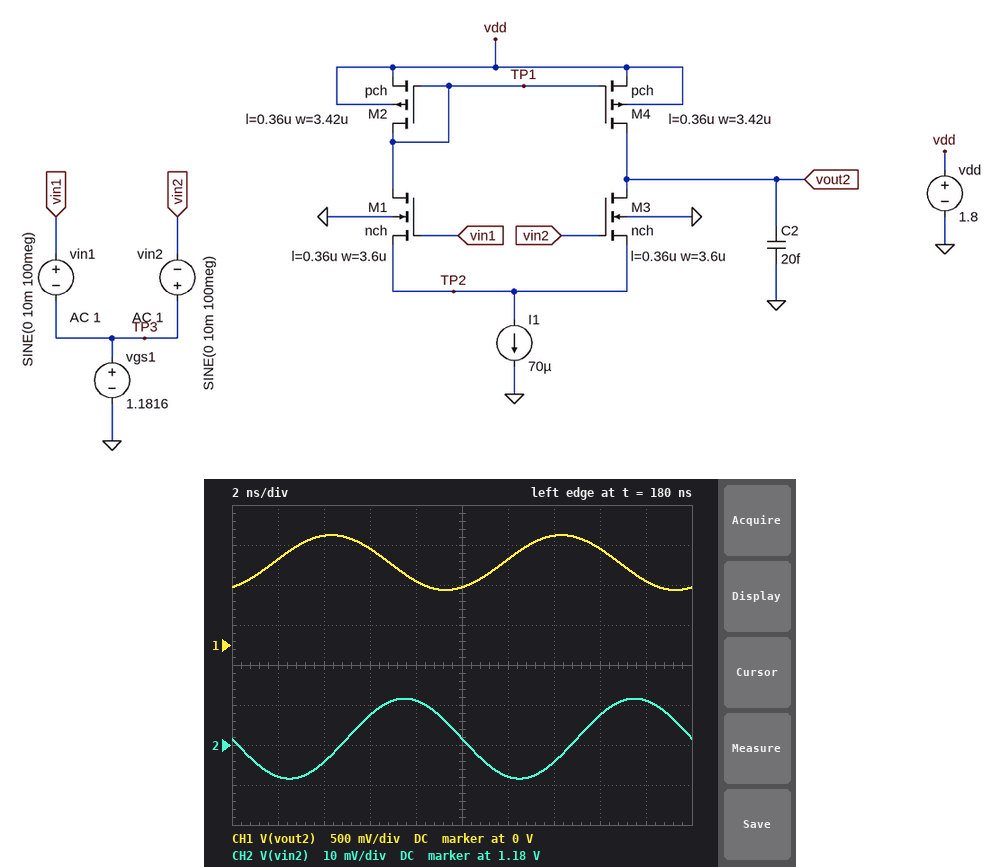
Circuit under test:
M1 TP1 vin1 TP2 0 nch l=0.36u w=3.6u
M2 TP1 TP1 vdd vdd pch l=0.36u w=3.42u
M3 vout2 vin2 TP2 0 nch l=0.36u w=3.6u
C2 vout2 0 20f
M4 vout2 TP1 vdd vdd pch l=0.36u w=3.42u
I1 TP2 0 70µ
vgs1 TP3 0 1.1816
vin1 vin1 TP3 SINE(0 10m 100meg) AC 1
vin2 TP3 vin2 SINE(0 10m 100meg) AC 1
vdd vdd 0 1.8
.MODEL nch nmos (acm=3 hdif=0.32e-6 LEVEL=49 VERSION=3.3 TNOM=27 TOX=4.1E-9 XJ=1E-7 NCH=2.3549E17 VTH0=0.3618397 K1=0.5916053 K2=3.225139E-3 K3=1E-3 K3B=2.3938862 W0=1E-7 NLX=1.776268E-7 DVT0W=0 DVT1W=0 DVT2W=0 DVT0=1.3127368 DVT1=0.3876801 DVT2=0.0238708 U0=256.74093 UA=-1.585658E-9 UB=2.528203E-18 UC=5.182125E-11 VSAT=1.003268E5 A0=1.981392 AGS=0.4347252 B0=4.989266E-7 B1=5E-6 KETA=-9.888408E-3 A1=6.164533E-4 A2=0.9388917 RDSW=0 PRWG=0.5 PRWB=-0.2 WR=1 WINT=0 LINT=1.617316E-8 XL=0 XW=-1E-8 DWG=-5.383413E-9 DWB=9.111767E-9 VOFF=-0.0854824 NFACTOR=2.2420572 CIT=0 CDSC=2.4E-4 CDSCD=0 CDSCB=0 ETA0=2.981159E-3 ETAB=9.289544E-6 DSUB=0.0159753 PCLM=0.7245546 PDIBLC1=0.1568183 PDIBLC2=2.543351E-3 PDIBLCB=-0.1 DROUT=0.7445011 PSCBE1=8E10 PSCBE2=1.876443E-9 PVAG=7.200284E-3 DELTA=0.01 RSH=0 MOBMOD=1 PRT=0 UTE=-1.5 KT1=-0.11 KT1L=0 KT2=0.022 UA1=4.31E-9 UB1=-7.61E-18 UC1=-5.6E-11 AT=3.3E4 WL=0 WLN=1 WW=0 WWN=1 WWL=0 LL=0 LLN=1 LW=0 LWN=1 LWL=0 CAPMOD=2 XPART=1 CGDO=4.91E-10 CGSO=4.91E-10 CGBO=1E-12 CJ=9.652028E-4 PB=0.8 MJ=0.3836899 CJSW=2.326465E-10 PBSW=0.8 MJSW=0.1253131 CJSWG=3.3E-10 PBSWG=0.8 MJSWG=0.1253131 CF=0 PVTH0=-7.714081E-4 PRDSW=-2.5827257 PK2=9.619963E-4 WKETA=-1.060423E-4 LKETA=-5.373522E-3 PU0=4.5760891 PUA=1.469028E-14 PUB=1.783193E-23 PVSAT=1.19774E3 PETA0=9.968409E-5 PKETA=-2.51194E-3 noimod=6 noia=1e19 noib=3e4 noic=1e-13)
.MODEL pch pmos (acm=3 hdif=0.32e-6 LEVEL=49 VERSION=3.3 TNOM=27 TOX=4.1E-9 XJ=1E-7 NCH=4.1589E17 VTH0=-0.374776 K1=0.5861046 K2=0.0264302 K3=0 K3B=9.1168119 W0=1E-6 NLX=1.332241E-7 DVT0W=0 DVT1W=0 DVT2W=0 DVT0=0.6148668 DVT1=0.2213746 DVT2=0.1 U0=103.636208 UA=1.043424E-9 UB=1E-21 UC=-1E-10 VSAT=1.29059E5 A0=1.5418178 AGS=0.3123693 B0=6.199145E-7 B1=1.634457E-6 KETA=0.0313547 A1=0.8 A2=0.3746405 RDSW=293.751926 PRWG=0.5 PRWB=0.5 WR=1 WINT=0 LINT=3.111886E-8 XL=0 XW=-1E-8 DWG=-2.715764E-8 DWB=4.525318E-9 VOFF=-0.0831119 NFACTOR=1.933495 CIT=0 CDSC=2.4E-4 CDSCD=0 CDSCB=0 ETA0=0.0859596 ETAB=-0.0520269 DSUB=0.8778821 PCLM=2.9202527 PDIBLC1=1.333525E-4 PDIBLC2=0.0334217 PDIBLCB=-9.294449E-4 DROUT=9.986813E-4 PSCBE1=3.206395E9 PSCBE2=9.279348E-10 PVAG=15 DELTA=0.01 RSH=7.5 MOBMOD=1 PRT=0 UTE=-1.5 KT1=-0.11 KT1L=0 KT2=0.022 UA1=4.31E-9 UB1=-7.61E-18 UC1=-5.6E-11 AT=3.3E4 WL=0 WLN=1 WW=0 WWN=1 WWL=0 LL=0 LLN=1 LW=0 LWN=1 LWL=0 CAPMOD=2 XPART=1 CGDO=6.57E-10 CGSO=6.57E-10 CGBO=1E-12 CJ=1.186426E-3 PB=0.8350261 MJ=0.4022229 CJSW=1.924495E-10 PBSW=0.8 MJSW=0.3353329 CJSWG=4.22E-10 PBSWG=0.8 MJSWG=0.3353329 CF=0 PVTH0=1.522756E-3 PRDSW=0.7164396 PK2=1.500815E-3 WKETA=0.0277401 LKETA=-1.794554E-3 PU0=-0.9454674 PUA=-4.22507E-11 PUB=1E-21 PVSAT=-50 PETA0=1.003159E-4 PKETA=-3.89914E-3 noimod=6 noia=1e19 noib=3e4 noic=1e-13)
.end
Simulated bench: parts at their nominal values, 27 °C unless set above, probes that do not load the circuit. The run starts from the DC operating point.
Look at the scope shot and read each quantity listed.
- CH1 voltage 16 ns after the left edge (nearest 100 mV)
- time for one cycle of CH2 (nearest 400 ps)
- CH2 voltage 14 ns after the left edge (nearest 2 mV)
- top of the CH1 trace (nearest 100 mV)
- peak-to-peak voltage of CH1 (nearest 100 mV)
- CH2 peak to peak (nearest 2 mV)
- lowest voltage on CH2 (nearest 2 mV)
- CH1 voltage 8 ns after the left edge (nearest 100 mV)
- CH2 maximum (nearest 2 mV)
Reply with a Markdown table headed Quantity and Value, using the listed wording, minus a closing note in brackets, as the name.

| Quantity | Value |
|---|---|
| CH1 voltage 16 ns after the left edge | 1.2 V |
| time for one cycle of CH2 | 10.0 ns |
| CH2 voltage 14 ns after the left edge | 1.176 V |
| top of the CH1 trace | 1.4 V |
| peak-to-peak voltage of CH1 | 700 mV |
| CH2 peak to peak | 20 mV |
| lowest voltage on CH2 | 1.172 V |
| CH1 voltage 8 ns after the left edge | 800 mV |
| CH2 maximum | 1.192 V |
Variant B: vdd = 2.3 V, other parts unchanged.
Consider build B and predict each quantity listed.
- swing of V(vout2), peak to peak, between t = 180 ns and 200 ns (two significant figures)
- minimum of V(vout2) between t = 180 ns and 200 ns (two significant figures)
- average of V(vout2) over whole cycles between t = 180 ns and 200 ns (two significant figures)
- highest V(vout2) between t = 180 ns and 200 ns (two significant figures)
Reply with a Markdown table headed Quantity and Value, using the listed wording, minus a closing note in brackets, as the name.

| Quantity | Value |
|---|---|
| swing of V(vout2), peak to peak, between t = 180 ns and 200 ns | 710 mV |
| minimum of V(vout2) between t = 180 ns and 200 ns | 1.2 V |
| average of V(vout2) over whole cycles between t = 180 ns and 200 ns | 1.5 V |
| highest V(vout2) between t = 180 ns and 200 ns | 1.9 V |
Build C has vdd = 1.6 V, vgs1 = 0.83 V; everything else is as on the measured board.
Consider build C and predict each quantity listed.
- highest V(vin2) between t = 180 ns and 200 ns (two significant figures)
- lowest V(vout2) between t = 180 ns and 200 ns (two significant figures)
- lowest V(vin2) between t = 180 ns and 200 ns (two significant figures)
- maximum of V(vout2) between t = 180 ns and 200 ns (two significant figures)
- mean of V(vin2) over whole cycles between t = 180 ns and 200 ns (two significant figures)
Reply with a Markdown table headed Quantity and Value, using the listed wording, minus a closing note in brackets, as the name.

| Quantity | Value |
|---|---|
| highest V(vin2) between t = 180 ns and 200 ns | 840 mV |
| lowest V(vout2) between t = 180 ns and 200 ns | 480 mV |
| lowest V(vin2) between t = 180 ns and 200 ns | 820 mV |
| maximum of V(vout2) between t = 180 ns and 200 ns | 1.2 V |
| mean of V(vin2) over whole cycles between t = 180 ns and 200 ns | 830 mV |
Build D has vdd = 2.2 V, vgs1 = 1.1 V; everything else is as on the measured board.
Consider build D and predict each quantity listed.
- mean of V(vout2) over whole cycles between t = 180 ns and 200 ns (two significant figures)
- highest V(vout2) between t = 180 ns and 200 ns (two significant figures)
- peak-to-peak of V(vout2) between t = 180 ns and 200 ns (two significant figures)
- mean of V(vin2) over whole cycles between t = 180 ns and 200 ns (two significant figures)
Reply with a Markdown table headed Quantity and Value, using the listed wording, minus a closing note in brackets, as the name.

| Quantity | Value |
|---|---|
| mean of V(vout2) over whole cycles between t = 180 ns and 200 ns | 1.4 V |
| highest V(vout2) between t = 180 ns and 200 ns | 1.8 V |
| peak-to-peak of V(vout2) between t = 180 ns and 200 ns | 710 mV |
| mean of V(vin2) over whole cycles between t = 180 ns and 200 ns | 1.1 V |
